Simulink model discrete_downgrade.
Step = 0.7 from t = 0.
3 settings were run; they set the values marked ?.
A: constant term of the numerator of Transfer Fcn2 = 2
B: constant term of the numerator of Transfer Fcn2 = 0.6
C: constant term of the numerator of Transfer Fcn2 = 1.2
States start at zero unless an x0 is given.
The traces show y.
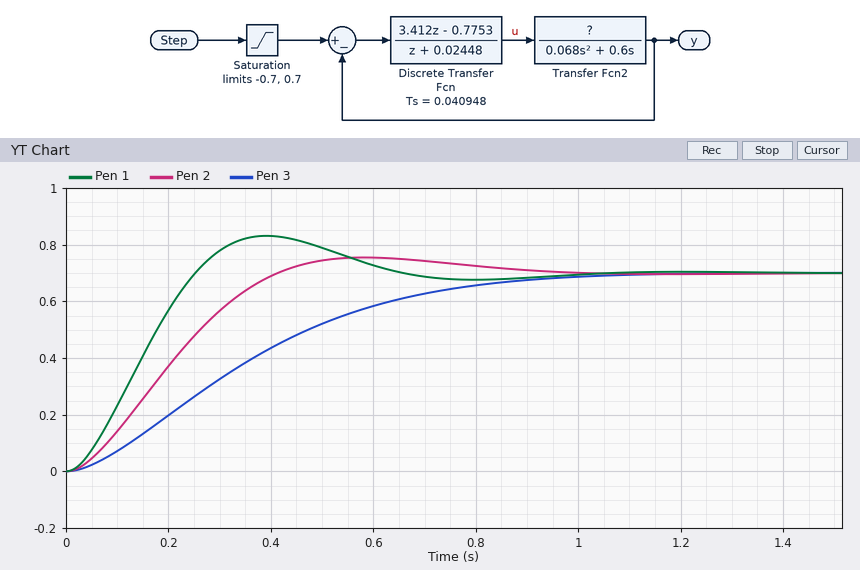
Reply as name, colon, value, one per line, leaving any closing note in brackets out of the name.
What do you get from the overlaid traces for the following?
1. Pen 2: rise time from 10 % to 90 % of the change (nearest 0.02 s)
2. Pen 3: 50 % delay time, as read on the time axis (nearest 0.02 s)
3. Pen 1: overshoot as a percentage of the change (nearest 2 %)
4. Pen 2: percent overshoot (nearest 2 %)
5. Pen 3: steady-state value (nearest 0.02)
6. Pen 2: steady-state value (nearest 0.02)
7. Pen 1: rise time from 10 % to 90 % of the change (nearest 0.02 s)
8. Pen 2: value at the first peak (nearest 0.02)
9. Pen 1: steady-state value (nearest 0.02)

Pen 2: rise time from 10 % to 90 % of the change: 0.28 s
Pen 3: 50 % delay time, as read on the time axis: 0.32 s
Pen 1: overshoot as a percentage of the change: 18 %
Pen 2: percent overshoot: 8 %
Pen 3: steady-state value: 0.70
Pen 2: steady-state value: 0.70
Pen 1: rise time from 10 % to 90 % of the change: 0.18 s
Pen 2: value at the first peak: 0.76
Pen 1: steady-state value: 0.70
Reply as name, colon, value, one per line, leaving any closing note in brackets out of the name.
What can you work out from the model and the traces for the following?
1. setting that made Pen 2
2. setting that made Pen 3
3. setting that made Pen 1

setting that made Pen 2: C
setting that made Pen 3: B
setting that made Pen 1: A
